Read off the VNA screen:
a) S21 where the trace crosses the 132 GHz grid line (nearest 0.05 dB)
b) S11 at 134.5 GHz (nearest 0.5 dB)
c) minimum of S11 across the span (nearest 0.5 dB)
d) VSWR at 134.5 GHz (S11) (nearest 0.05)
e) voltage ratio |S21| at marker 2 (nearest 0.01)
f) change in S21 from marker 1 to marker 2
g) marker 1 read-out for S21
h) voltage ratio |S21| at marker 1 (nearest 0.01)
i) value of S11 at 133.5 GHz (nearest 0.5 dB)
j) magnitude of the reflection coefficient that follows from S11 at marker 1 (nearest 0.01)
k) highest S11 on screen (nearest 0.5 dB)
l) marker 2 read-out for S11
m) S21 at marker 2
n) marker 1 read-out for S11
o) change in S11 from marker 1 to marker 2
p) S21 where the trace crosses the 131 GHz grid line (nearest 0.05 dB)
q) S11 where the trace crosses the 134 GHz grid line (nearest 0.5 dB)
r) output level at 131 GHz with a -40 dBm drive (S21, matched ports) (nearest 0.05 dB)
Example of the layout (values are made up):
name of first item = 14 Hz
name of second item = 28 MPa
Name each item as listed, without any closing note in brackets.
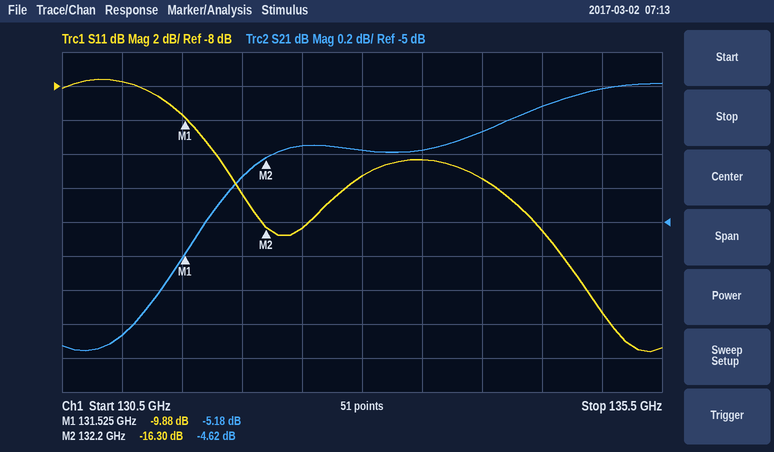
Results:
S21 where the trace crosses the 132 GHz grid line = -4.75 dB
S11 at 134.5 GHz = -16.5 dB
minimum of S11 across the span = -23.5 dB
VSWR at 134.5 GHz (S11) = 1.35
voltage ratio |S21| at marker 2 = 0.59
change in S21 from marker 1 to marker 2 = 0.56 dB
marker 1 read-out for S21 = -5.18 dB
voltage ratio |S21| at marker 1 = 0.55
value of S11 at 133.5 GHz = -12.5 dB
magnitude of the reflection coefficient that follows from S11 at marker 1 = 0.32
highest S11 on screen = -7.5 dB
marker 2 read-out for S11 = -16.30 dB
S21 at marker 2 = -4.62 dB
marker 1 read-out for S11 = -9.88 dB
change in S11 from marker 1 to marker 2 = -6.42 dB
S21 where the trace crosses the 131 GHz grid line = -5.65 dB
S11 where the trace crosses the 134 GHz grid line = -13.5 dB
output level at 131 GHz with a -40 dBm drive (S21, matched ports) = -45.65 dBm
